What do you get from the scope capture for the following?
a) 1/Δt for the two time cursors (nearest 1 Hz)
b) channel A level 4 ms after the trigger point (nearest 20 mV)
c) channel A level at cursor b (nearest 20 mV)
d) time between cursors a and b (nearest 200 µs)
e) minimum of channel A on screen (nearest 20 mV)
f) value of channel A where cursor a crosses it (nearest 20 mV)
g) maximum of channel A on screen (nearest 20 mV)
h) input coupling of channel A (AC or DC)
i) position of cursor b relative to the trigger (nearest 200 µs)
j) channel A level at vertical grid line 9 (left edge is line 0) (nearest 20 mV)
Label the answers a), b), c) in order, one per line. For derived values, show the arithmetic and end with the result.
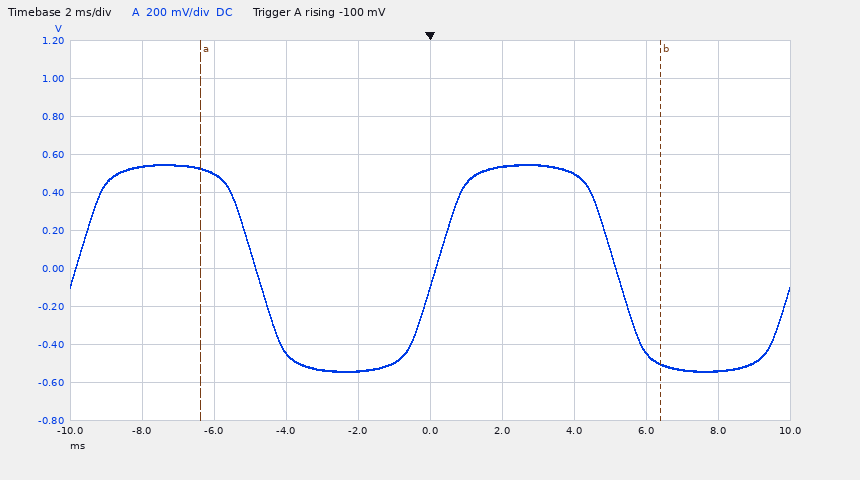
a) 1 / 12.8 ms ≈ 78 Hz
b) 500 mV
c) -500 mV
d) 12.8 ms
e) -540 mV
f) 520 mV
g) 540 mV
h) DC
i) +6.4 ms
j) -540 mV
